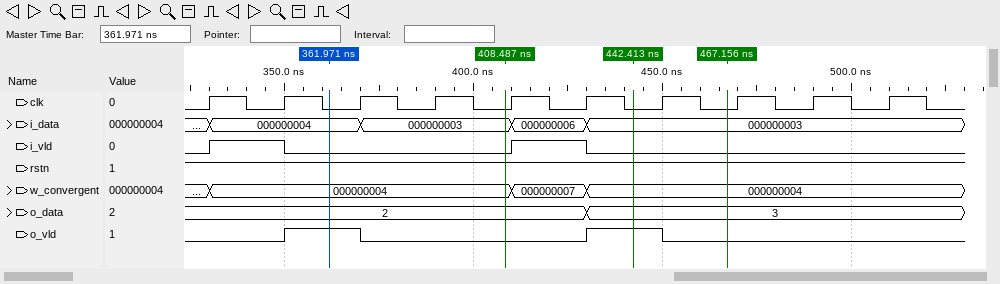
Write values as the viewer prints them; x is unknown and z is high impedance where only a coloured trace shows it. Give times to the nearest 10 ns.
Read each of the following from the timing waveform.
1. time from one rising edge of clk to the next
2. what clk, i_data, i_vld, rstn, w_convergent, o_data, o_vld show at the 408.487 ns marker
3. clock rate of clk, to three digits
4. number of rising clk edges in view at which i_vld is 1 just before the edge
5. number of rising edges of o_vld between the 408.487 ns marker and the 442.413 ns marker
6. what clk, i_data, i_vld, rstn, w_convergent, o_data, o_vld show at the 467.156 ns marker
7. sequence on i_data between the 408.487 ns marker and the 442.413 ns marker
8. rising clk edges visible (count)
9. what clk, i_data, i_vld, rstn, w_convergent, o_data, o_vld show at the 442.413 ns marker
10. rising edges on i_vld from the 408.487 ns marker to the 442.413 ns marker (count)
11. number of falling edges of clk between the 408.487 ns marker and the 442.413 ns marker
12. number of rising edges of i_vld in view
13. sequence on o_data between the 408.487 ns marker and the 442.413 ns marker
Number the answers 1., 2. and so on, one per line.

1. 20 ns
2. clk=0, i_data=000000003, i_vld=0, rstn=1, w_convergent=000000004, o_data=2, o_vld=0
3. 50.0 MHz
4. 2
5. 1
6. clk=0, i_data=000000003, i_vld=0, rstn=1, w_convergent=000000004, o_data=3, o_vld=0
7. 000000003, 000000006, 000000003
8. 10
9. clk=0, i_data=000000003, i_vld=0, rstn=1, w_convergent=000000004, o_data=3, o_vld=1
10. 1
11. 2
12. 2
13. 2, 3
